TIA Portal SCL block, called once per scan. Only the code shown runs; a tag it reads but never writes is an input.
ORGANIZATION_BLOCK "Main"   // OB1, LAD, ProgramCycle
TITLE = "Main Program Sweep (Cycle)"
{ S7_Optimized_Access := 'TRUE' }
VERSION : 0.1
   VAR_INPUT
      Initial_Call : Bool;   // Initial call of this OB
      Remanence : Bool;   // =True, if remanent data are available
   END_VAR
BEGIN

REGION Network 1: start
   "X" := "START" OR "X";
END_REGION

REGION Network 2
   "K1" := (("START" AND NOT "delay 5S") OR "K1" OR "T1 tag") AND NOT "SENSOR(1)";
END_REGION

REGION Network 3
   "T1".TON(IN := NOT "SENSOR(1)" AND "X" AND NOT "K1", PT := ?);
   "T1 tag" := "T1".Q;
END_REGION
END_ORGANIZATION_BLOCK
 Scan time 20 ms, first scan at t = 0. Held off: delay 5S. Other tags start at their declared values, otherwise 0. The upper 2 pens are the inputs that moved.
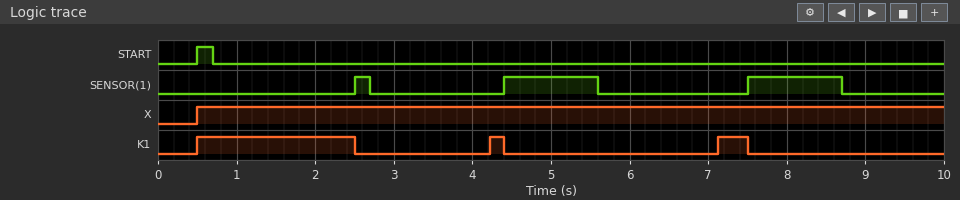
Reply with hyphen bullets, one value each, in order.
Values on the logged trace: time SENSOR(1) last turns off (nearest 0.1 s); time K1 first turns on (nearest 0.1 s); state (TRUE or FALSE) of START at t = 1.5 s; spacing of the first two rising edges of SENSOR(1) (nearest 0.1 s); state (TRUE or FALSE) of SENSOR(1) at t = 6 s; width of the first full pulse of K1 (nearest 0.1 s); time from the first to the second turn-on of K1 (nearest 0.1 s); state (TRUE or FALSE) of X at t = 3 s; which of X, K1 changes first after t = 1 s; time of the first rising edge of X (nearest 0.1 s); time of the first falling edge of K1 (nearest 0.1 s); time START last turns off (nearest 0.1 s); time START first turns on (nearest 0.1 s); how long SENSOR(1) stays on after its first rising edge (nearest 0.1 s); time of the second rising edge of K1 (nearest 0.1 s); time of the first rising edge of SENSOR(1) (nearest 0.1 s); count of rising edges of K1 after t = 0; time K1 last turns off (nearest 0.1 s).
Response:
- 8.7 s
- 0.5 s
- FALSE
- 1.9 s
- FALSE
- 2.0 s
- 3.7 s
- TRUE
- K1
- 0.5 s
- 2.5 s
- 0.7 s
- 0.5 s
- 0.2 s
- 4.2 s
- 2.5 s
- 3
- 7.5 s
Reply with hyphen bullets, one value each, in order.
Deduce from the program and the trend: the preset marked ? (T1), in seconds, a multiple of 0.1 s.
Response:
- 1.5 s
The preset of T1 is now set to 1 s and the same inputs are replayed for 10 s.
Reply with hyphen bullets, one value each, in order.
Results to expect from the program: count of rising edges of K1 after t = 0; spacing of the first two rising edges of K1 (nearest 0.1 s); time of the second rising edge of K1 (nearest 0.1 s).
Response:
- 4
- 3.2 s
- 3.7 s
